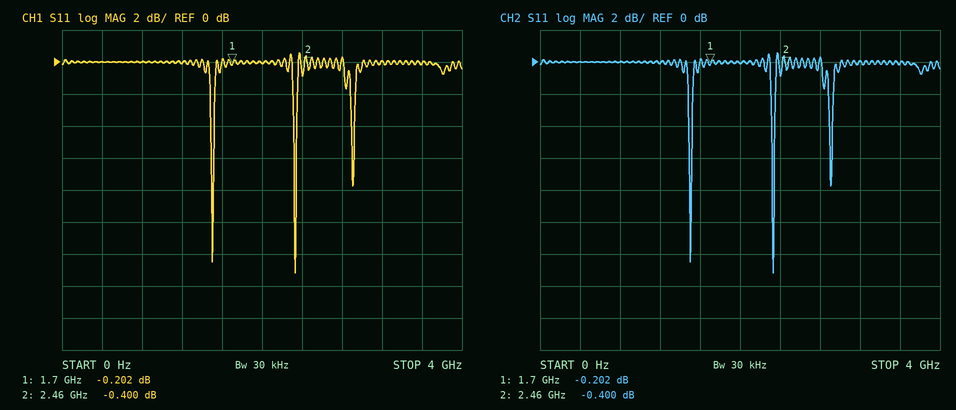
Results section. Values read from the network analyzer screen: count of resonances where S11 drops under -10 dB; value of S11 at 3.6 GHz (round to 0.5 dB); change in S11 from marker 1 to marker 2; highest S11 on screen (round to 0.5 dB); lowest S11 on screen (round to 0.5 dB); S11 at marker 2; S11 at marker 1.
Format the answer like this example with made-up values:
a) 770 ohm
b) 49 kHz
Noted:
a) 2
b) 0.0 dB
c) -0.198 dB
d) 0.5 dB
e) -13.0 dB
f) -0.400 dB
g) -0.202 dB
